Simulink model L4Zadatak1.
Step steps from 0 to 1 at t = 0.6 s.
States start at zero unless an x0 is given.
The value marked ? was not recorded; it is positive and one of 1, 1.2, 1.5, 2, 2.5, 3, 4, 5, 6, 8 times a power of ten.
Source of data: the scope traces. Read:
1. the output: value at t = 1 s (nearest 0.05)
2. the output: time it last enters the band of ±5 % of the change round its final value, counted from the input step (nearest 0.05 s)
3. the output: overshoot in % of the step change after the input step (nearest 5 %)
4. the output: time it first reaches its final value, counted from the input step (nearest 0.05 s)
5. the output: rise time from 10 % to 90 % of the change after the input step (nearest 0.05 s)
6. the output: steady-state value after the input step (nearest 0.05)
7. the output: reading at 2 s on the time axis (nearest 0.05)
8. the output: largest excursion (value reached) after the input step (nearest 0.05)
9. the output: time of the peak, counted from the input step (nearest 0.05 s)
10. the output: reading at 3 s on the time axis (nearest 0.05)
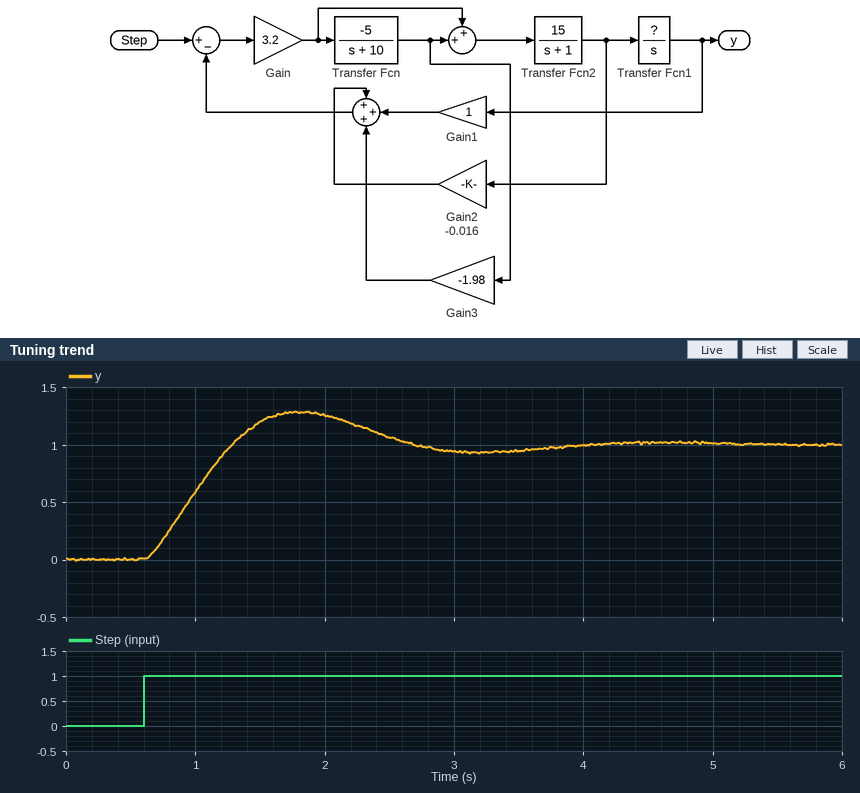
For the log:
0.60
2.95 s
30 %
0.70 s
0.50 s
1.00
1.25
1.30
1.20 s
0.95
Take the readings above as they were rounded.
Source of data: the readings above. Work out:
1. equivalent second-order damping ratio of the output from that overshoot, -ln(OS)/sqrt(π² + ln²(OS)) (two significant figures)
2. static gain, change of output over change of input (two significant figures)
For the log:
0.36
1.0
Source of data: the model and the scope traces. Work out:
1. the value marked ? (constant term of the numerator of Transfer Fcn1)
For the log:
1
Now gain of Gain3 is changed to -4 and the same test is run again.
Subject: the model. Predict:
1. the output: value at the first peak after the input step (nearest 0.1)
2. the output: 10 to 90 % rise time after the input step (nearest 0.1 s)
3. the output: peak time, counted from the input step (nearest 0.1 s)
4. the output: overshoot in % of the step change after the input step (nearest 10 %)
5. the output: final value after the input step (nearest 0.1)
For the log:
1.2
0.8 s
1.7 s
20 %
1.0
